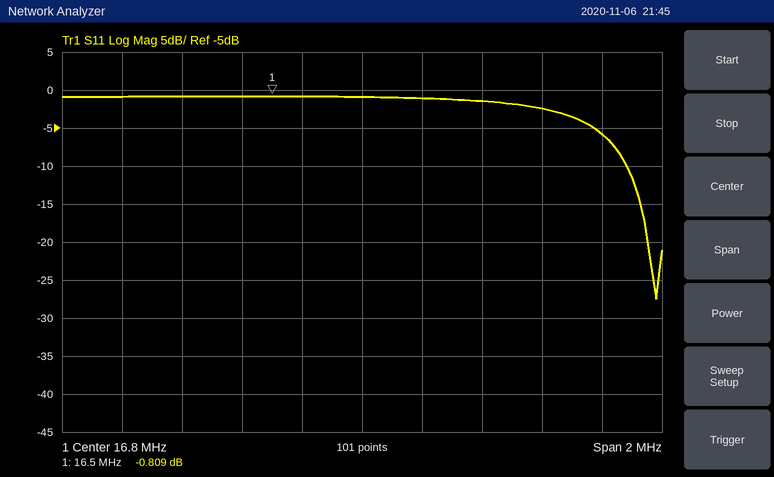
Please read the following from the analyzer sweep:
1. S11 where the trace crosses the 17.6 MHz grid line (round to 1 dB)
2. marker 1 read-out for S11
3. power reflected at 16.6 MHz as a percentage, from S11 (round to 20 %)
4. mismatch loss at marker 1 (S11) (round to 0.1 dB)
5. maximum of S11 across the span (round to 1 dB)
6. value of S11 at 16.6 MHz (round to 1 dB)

-6 dB
-0.809 dB
80 %
7.7 dB
-1 dB
-1 dB
